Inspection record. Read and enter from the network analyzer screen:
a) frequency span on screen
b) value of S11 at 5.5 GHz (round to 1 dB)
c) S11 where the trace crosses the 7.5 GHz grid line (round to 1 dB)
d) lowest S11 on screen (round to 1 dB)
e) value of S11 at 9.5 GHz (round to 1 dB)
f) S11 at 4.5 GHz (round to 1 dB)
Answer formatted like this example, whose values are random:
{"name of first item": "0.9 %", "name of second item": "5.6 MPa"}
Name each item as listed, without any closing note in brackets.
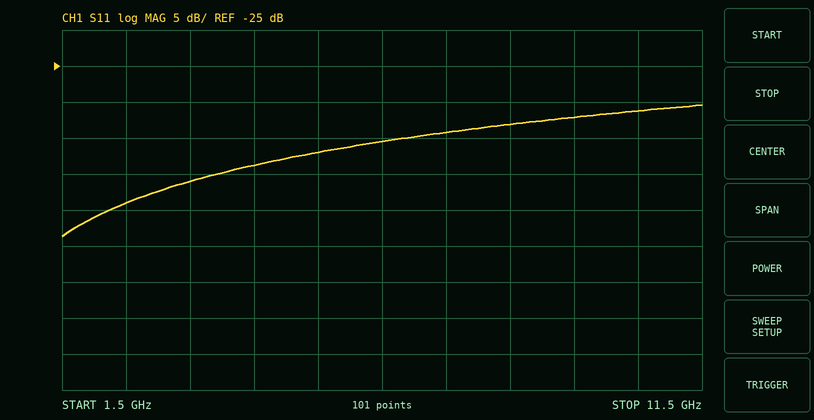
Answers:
{"frequency span on screen": "10 GHz", "value of S11 at 5.5 GHz": "-37 dB", "S11 where the trace crosses the 7.5 GHz grid line": "-34 dB", "lowest S11 on screen": "-49 dB", "value of S11 at 9.5 GHz": "-32 dB", "S11 at 4.5 GHz": "-39 dB"}
